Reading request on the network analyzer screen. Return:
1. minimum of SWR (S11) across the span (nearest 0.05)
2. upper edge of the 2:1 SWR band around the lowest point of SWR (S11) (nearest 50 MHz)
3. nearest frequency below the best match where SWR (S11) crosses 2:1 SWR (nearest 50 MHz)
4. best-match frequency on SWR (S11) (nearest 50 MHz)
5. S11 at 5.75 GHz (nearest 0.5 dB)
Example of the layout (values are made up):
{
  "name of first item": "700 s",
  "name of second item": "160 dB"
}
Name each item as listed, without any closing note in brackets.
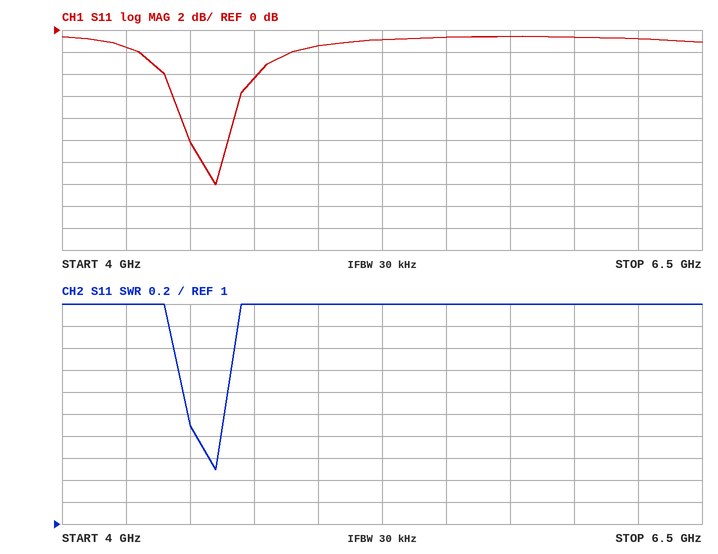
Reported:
{
  "minimum of SWR (S11) across the span": "1.50",
  "upper edge of the 2:1 SWR band around the lowest point of SWR (S11)": "4.65 GHz",
  "nearest frequency below the best match where SWR (S11) crosses 2:1 SWR": "4.50 GHz",
  "best-match frequency on SWR (S11)": "4.60 GHz",
  "S11 at 5.75 GHz": "-0.5 dB"
}
